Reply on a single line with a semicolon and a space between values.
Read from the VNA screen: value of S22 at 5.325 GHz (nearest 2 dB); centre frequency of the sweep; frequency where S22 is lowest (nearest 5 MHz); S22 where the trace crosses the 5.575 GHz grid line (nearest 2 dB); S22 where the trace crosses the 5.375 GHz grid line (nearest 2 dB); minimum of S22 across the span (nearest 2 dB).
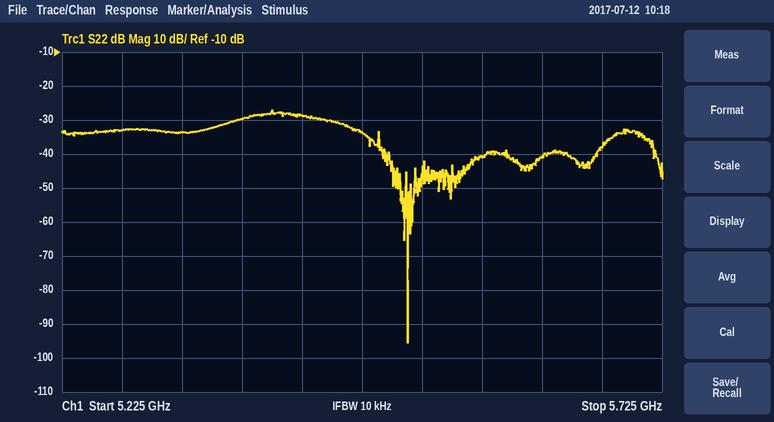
-34 dB; 5.475 GHz; 5.515 GHz; -40 dB; -30 dB; -96 dB
